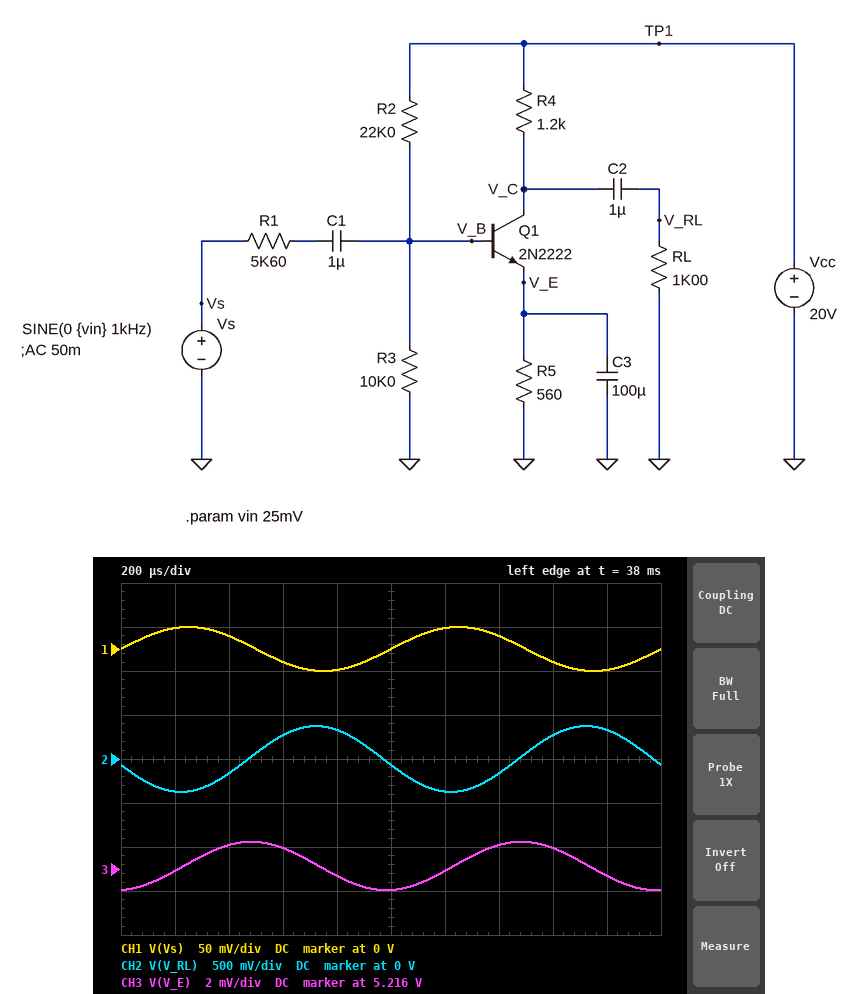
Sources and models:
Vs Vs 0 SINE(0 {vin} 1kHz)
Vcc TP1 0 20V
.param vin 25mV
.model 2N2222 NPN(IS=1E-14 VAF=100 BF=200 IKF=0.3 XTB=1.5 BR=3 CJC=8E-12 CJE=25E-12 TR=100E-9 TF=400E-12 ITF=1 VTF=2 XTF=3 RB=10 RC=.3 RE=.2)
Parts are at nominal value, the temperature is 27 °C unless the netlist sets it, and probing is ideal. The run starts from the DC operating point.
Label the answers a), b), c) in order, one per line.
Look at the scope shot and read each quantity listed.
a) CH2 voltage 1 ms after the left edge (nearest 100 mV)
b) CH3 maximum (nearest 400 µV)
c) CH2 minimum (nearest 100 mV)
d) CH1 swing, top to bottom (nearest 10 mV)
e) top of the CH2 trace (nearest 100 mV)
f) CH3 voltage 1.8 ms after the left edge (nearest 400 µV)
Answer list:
a) -100 mV
b) 5.2172 V
c) -400 mV
d) 50 mV
e) 400 mV
f) 5.2156 V
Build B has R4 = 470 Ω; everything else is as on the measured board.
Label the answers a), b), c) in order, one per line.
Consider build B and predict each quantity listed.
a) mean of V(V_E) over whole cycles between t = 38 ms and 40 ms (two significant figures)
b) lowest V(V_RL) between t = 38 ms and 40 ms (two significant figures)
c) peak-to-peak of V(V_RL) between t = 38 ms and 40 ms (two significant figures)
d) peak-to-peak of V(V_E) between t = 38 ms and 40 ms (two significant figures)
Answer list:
a) 5.2 V
b) -240 mV
c) 470 mV
d) 2.4 mV
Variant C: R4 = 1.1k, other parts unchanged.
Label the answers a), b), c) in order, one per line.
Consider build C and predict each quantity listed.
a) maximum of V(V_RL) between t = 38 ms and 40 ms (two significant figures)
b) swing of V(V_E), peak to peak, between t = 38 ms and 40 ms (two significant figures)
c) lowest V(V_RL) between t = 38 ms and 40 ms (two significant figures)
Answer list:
a) 360 mV
b) 2.2 mV
c) -360 mV
